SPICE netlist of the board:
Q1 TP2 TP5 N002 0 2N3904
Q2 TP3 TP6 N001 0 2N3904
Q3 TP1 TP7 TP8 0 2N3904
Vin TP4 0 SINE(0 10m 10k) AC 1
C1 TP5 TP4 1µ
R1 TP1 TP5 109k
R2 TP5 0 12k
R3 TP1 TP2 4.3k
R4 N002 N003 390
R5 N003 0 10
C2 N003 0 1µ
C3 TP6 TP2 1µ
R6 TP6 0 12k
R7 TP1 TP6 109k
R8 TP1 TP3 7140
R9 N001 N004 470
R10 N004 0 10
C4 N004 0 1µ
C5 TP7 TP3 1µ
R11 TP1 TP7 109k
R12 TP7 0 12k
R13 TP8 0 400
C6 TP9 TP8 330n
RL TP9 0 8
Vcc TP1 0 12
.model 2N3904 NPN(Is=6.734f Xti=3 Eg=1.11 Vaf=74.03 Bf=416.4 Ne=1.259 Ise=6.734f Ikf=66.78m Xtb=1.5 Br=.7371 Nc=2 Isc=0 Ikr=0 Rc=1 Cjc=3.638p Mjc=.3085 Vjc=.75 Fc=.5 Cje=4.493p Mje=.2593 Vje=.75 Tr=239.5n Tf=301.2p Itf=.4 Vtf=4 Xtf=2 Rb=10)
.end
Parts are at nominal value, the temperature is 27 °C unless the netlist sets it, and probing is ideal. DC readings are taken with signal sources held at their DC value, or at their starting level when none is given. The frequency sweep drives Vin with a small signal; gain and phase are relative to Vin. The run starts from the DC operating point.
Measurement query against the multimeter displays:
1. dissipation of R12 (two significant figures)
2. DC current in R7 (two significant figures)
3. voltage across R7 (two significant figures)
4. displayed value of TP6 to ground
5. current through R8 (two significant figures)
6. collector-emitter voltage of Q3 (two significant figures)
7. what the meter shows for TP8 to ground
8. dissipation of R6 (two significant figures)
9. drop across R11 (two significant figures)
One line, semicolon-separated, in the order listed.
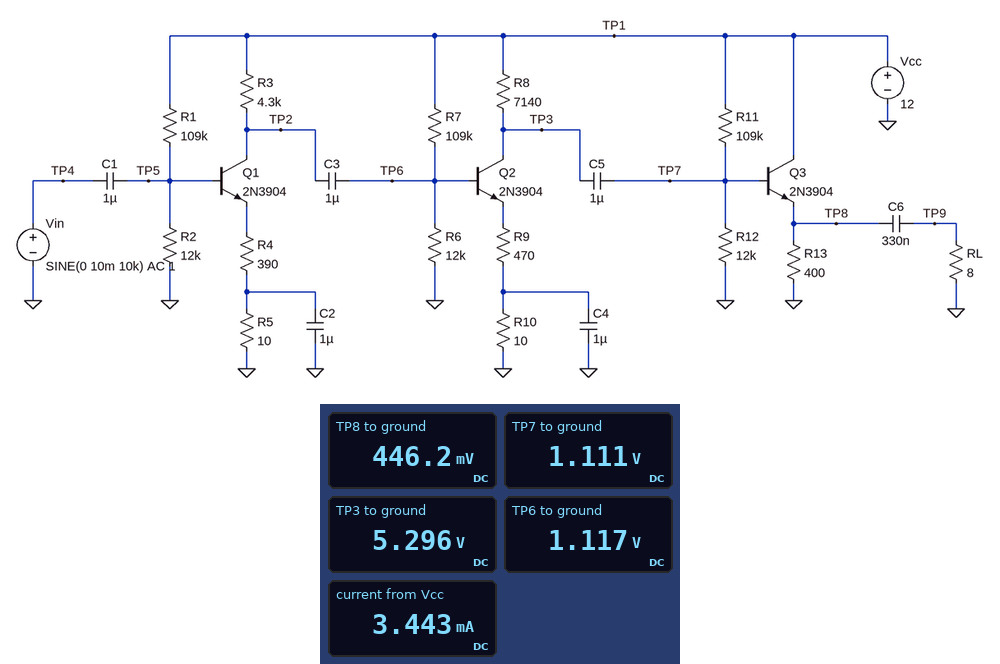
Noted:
100 µW; 100 µA; 11 V; 1.117 V; 940 µA; 12 V; 446.2 mV; 100 µW; 11 V
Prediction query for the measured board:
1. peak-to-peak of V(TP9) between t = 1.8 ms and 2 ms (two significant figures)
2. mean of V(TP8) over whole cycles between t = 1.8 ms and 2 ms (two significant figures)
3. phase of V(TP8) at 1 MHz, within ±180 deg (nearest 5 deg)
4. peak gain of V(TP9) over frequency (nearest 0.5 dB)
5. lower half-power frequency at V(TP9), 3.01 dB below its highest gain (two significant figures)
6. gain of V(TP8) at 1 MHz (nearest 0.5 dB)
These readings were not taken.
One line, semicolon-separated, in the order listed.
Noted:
62 mV; 720 mV; -35 deg; 18.5 dB; 10 kHz; 17.5 dB
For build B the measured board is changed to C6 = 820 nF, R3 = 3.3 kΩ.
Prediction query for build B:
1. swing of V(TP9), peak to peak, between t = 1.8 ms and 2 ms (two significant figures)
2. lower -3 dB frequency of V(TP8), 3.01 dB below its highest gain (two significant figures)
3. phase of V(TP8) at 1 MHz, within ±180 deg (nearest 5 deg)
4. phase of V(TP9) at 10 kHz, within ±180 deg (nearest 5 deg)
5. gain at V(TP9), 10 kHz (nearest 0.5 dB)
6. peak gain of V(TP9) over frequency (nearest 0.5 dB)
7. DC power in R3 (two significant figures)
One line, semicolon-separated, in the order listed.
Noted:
58 mV; 26 Hz; -30 deg; 20 deg; 16.0 dB; 17.0 dB; 4.0 mW
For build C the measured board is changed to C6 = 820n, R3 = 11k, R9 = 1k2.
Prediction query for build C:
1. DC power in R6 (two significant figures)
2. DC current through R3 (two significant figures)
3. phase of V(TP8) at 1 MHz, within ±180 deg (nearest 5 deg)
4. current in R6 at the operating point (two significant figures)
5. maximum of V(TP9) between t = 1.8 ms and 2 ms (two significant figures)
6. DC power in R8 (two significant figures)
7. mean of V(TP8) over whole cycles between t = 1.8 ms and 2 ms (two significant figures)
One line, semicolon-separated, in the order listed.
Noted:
110 µW; 1.0 mA; -50 deg; 96 µA; 21 mV; 1.3 mW; 480 mV
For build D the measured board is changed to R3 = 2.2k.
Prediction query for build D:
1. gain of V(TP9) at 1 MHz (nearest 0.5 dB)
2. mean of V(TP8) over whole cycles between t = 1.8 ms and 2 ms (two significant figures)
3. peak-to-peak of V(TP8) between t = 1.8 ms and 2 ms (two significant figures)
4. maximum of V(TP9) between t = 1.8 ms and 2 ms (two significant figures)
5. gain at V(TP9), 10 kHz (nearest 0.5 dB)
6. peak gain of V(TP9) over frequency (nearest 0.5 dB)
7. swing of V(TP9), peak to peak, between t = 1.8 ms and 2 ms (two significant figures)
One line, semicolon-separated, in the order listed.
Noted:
13.5 dB; 580 mV; 260 mV; 31 mV; 11.0 dB; 14.0 dB; 44 mV
